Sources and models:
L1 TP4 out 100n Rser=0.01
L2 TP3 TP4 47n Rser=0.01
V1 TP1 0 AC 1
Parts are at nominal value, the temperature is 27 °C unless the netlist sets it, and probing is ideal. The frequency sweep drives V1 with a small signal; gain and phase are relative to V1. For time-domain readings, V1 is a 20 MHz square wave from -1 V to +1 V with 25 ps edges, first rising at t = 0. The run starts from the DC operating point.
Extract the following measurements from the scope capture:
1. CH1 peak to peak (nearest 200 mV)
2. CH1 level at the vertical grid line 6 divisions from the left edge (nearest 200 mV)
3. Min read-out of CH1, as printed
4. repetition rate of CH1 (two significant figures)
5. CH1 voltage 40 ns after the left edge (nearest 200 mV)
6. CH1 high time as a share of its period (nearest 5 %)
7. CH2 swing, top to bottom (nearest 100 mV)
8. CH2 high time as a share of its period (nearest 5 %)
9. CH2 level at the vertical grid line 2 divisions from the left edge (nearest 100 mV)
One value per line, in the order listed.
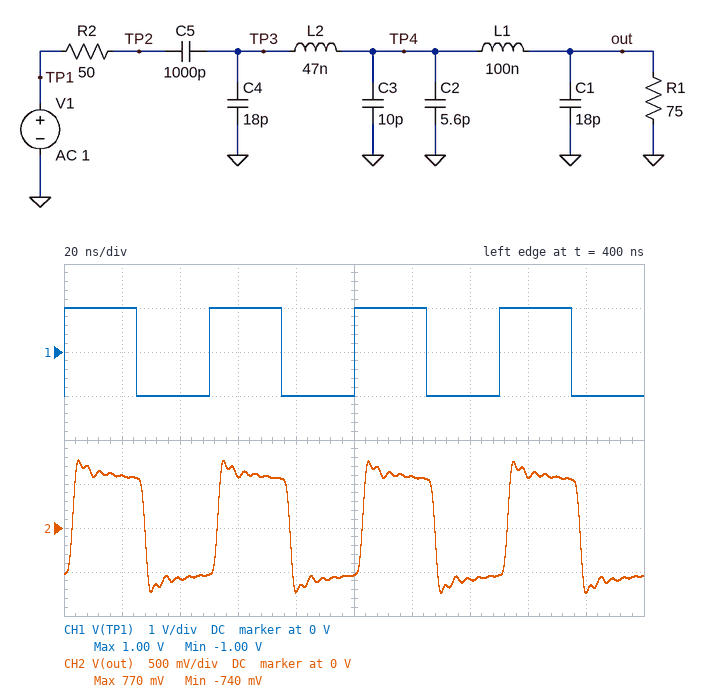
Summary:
2.0 V
1.0 V
-1.00 V
20 MHz
-1.0 V
50 %
1.5 V
50 %
-600 mV
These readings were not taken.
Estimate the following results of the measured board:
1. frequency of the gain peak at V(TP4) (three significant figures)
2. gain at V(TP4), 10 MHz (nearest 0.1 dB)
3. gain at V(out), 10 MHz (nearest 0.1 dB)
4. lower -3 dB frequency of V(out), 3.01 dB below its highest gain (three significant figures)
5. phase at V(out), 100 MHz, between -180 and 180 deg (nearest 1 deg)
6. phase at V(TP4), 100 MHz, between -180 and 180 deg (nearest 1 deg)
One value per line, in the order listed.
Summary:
261 MHz
-4.6 dB
-4.6 dB
1.31 MHz
-104 deg
-33 deg
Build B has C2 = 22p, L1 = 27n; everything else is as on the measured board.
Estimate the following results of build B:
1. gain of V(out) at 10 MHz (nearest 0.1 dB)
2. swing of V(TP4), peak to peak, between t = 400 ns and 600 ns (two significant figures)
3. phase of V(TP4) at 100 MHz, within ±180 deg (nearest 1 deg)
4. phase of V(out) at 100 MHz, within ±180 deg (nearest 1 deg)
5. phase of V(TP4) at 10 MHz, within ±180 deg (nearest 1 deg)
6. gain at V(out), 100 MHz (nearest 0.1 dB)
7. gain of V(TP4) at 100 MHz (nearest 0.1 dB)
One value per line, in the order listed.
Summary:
-4.7 dB
1.3 V
-68 deg
-84 deg
-1 deg
-5.4 dB
-6.9 dB
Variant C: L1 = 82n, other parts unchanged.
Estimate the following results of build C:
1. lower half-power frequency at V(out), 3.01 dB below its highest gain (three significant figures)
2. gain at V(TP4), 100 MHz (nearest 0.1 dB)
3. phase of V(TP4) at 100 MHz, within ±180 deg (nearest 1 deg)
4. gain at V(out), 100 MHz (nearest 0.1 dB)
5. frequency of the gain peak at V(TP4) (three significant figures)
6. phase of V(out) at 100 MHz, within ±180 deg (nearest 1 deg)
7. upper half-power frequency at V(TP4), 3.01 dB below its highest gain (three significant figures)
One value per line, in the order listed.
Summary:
1.32 MHz
-6.2 dB
-38 deg
-4.3 dB
269 MHz
-96 deg
290 MHz
